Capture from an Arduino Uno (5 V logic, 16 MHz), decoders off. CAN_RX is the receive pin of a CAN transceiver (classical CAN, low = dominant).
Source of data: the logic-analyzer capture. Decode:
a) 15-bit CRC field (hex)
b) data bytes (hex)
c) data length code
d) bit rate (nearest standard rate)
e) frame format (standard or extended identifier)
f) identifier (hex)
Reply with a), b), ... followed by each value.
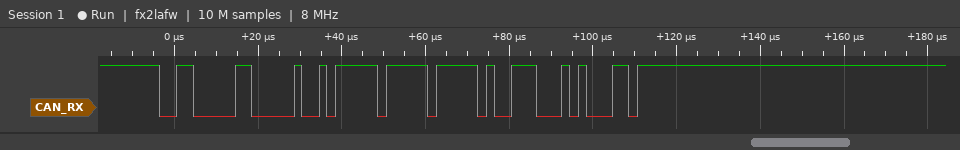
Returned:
a) 0x1C51
b) FF FF
c) 2
d) 500 kbit/s
e) standard
f) 0x304
